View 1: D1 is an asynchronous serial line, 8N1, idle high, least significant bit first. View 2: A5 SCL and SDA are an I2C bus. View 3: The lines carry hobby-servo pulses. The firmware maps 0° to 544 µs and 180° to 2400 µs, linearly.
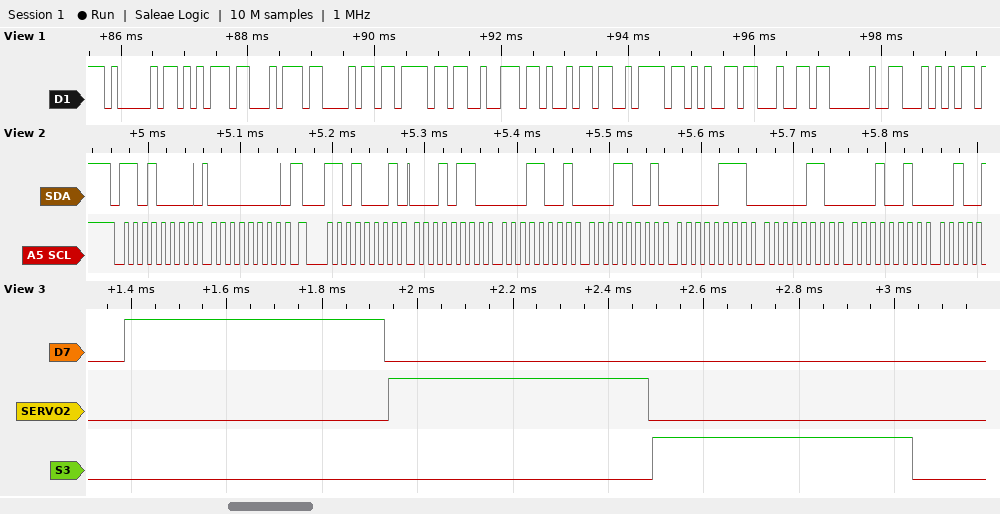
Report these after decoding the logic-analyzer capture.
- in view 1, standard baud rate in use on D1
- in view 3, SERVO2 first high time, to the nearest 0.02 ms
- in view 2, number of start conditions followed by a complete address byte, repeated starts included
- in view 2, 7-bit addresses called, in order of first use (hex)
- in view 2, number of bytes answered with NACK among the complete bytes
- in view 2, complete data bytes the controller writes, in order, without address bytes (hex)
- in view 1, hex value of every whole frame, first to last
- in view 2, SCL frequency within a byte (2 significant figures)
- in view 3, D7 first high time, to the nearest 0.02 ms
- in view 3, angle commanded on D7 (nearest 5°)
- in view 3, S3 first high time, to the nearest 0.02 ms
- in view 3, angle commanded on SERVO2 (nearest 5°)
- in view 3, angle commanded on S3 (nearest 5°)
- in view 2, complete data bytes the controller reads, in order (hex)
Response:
9600 baud
0.54 ms
2
0x68
0
00
0x41 0x75 0x74 0x68 0x6F 0x72 0x69 0x7A 0x65 0x64 0x20 0x54
100 kHz
0.54 ms
0°
0.54 ms
0°
0°
16 19 19 07 06 12
